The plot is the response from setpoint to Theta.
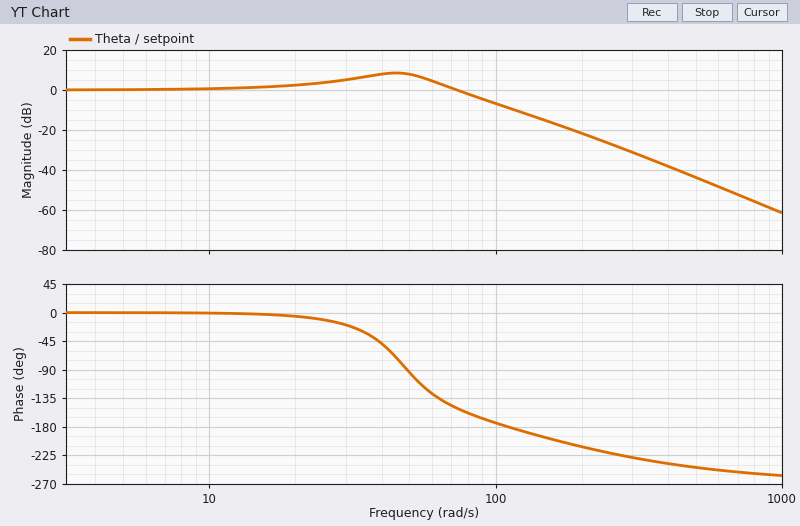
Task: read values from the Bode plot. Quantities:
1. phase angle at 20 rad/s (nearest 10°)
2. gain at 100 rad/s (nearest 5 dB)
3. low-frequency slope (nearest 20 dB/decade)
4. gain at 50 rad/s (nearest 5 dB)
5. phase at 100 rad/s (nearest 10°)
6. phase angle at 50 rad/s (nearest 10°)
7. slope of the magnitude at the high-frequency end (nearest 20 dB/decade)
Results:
-10°
-5 dB
0 dB/decade
10 dB
-170°
-90°
-60 dB/decade
